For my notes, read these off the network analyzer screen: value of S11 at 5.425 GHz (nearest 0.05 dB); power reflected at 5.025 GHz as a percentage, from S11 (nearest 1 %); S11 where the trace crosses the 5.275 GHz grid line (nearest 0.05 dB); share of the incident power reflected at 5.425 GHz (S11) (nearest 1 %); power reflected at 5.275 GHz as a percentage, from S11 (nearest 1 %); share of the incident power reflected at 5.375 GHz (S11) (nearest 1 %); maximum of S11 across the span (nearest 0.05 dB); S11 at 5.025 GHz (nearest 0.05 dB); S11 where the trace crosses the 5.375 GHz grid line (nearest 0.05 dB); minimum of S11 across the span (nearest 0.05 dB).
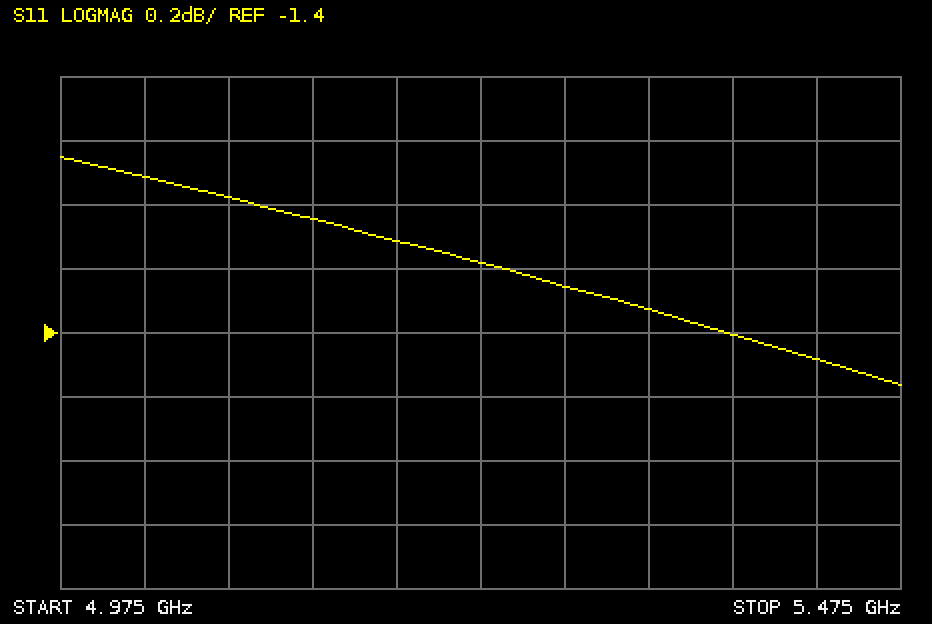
-1.50 dB
81 %
-1.25 dB
71 %
75 %
72 %
-0.85 dB
-0.90 dB
-1.40 dB
-1.55 dB
